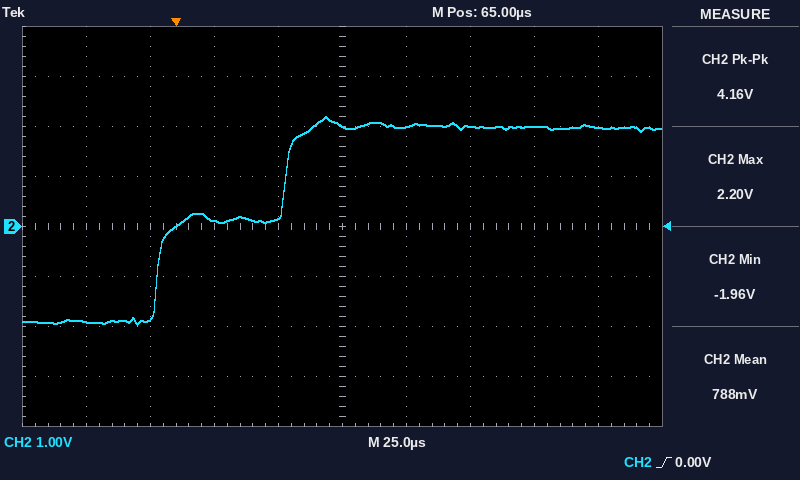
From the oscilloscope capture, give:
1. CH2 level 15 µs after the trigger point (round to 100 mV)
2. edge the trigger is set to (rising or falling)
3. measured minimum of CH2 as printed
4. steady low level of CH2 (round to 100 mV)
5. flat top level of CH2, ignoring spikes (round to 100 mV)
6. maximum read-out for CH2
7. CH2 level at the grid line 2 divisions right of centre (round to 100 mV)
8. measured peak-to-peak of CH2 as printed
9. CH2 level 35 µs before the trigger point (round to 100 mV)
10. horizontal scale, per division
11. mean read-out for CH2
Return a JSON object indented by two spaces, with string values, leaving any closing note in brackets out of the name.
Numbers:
{
  "CH2 level 15 µs after the trigger point": "100 mV",
  "edge the trigger is set to": "rising",
  "measured minimum of CH2 as printed": "-1.96 V",
  "steady low level of CH2": "-1.9 V",
  "flat top level of CH2, ignoring spikes": "2.0 V",
  "maximum read-out for CH2": "2.20 V",
  "CH2 level at the grid line 2 divisions right of centre": "2.0 V",
  "measured peak-to-peak of CH2 as printed": "4.16 V",
  "CH2 level 35 µs before the trigger point": "-1.9 V",
  "horizontal scale, per division": "25 µs",
  "mean read-out for CH2": "788 mV"
}
